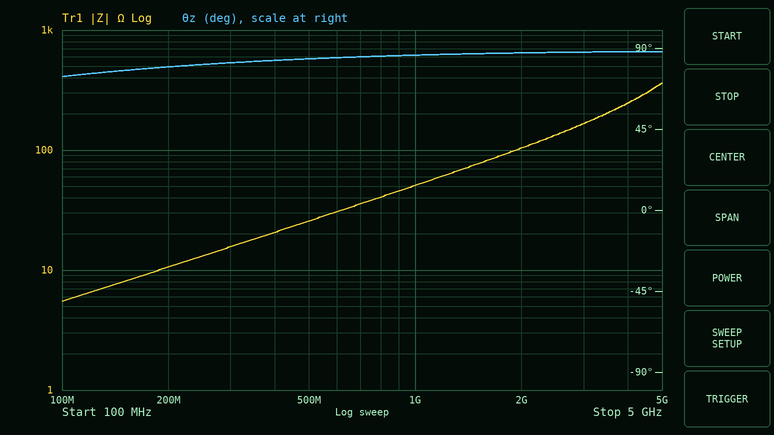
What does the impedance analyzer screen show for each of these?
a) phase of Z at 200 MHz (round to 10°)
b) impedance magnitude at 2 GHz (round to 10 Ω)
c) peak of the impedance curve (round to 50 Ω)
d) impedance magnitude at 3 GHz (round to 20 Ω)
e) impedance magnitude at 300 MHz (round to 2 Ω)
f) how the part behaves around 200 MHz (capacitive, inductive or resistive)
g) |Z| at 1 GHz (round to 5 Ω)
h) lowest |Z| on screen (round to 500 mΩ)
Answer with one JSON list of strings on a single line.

["80°", "100 Ω", "350 Ω", "160 Ω", "16 Ω", "inductive", "50 Ω", "5.5 Ω"]
